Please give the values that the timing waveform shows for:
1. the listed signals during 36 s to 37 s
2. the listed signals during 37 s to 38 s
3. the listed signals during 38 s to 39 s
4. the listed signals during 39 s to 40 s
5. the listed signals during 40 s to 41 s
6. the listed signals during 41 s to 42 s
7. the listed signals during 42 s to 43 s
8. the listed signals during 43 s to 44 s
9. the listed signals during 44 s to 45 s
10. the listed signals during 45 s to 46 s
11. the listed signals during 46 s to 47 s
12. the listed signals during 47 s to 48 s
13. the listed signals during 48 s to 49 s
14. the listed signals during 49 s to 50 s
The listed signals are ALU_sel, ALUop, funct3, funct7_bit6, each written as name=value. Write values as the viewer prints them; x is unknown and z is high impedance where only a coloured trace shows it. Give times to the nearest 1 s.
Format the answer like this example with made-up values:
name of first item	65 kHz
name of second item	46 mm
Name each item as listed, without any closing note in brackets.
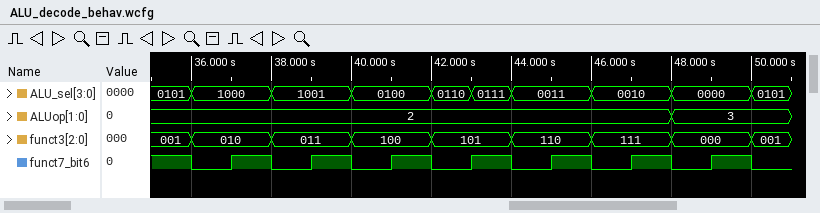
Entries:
the listed signals during 36 s to 37 s	ALU_sel=1000, ALUop=2, funct3=010, funct7_bit6=0
the listed signals during 37 s to 38 s	ALU_sel=1000, ALUop=2, funct3=010, funct7_bit6=1
the listed signals during 38 s to 39 s	ALU_sel=1001, ALUop=2, funct3=011, funct7_bit6=0
the listed signals during 39 s to 40 s	ALU_sel=1001, ALUop=2, funct3=011, funct7_bit6=1
the listed signals during 40 s to 41 s	ALU_sel=0100, ALUop=2, funct3=100, funct7_bit6=0
the listed signals during 41 s to 42 s	ALU_sel=0100, ALUop=2, funct3=100, funct7_bit6=1
the listed signals during 42 s to 43 s	ALU_sel=0110, ALUop=2, funct3=101, funct7_bit6=0
the listed signals during 43 s to 44 s	ALU_sel=0111, ALUop=2, funct3=101, funct7_bit6=1
the listed signals during 44 s to 45 s	ALU_sel=0011, ALUop=2, funct3=110, funct7_bit6=0
the listed signals during 45 s to 46 s	ALU_sel=0011, ALUop=2, funct3=110, funct7_bit6=1
the listed signals during 46 s to 47 s	ALU_sel=0010, ALUop=2, funct3=111, funct7_bit6=0
the listed signals during 47 s to 48 s	ALU_sel=0010, ALUop=2, funct3=111, funct7_bit6=1
the listed signals during 48 s to 49 s	ALU_sel=0000, ALUop=3, funct3=000, funct7_bit6=0
the listed signals during 49 s to 50 s	ALU_sel=0000, ALUop=3, funct3=000, funct7_bit6=1
